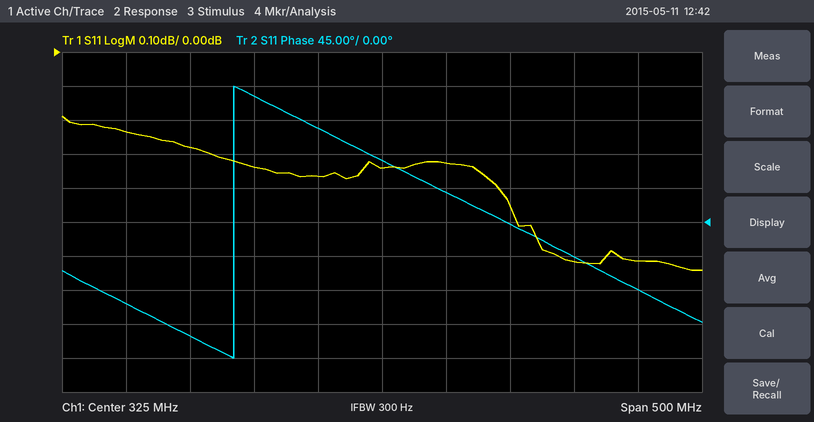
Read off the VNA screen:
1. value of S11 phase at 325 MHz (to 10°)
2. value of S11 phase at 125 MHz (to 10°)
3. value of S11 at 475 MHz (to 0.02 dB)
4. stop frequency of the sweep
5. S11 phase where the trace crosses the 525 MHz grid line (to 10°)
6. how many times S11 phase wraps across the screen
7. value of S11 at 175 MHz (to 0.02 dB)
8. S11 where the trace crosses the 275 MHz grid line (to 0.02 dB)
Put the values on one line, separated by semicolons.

80°; -110°; -0.62 dB; 575 MHz; -90°; 1; -0.28 dB; -0.36 dB
